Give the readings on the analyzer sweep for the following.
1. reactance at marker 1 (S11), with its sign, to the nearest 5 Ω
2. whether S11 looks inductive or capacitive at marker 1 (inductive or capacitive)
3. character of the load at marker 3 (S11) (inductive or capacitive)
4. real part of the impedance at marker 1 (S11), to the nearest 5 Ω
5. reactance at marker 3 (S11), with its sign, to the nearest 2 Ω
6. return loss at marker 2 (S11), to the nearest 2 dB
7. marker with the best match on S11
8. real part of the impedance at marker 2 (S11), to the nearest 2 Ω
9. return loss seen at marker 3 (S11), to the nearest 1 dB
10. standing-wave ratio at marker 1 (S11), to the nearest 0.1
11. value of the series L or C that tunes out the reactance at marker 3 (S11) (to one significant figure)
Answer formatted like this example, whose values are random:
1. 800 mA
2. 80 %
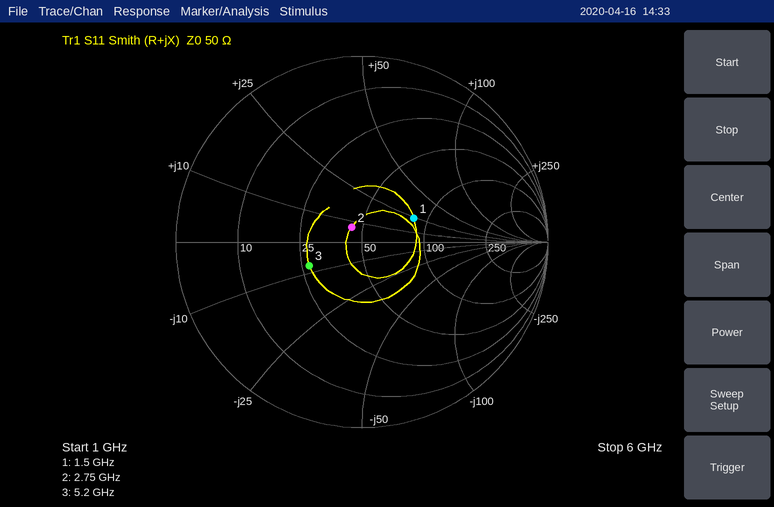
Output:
1. +25 Ω
2. inductive
3. capacitive
4. 85 Ω
5. -8 Ω
6. 20 dB
7. marker 2
8. 44 Ω
9. 10 dB
10. 1.9
11. 200 pH
